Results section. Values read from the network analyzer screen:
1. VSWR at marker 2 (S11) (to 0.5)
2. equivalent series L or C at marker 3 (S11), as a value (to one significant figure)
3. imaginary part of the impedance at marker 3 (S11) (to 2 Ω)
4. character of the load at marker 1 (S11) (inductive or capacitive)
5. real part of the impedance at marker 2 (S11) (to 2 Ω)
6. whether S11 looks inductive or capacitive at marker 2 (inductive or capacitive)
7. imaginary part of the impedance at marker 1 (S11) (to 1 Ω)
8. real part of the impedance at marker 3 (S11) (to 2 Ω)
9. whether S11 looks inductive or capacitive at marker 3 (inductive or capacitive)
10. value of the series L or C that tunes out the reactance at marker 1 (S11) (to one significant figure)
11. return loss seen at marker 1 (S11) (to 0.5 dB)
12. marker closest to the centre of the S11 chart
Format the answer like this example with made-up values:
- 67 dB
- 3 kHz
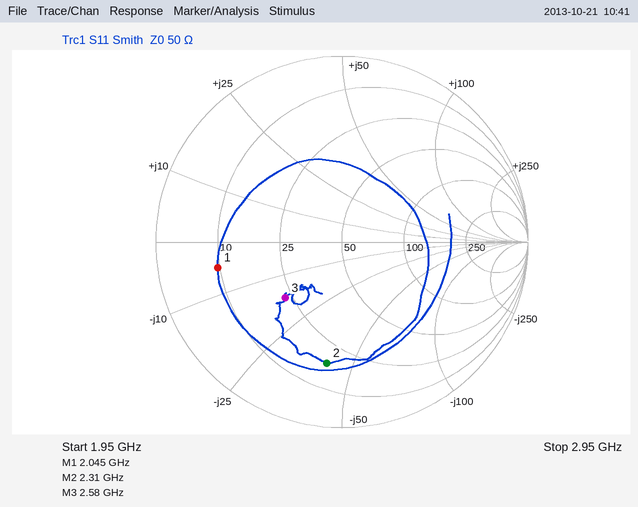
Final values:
- 5.0
- 4 pF
- -16 Ω
- capacitive
- 18 Ω
- capacitive
- -5 Ω
- 22 Ω
- capacitive
- 400 pH
- 3.5 dB
- marker 3
